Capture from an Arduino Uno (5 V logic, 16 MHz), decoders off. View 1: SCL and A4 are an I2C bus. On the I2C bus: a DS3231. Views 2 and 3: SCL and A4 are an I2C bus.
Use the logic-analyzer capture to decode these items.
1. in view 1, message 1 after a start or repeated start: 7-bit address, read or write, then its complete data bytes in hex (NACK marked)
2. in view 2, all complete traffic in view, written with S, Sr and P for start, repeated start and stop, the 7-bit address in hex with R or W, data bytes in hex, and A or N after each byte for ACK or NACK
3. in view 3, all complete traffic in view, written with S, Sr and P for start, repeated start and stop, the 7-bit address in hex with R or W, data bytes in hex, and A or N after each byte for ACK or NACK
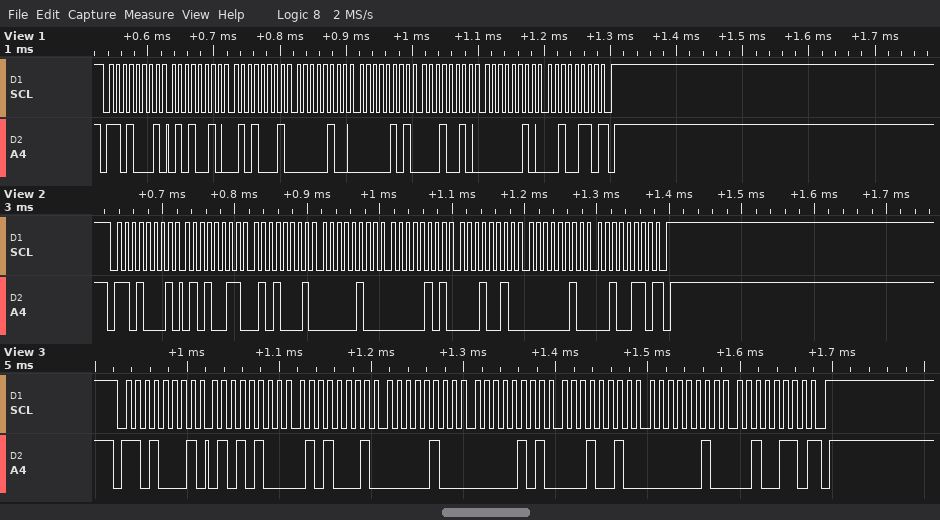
0x68 read: 52 51 04 05 12 02 26 NACK
S 68R A 53 A 51 A 04 A 05 A 12 A 02 A 26 N P
S 68R A 54 A 51 A 04 A 05 A 12 A 02 A 26 N P
